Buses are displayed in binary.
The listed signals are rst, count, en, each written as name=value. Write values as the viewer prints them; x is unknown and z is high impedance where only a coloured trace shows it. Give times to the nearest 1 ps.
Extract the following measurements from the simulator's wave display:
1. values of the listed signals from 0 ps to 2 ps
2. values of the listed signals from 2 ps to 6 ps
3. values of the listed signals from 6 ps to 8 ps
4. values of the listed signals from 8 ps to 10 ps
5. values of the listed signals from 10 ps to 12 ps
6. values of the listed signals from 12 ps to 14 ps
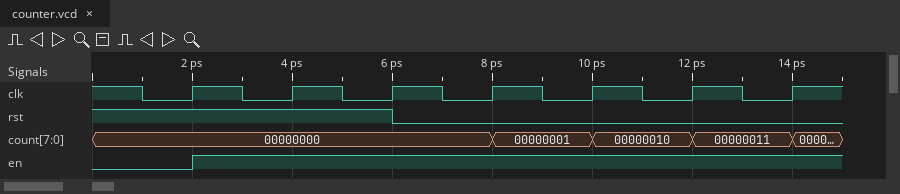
rst=1, count=00000000, en=0
rst=1, count=00000000, en=1
rst=0, count=00000000, en=1
rst=0, count=00000001, en=1
rst=0, count=00000010, en=1
rst=0, count=00000011, en=1
